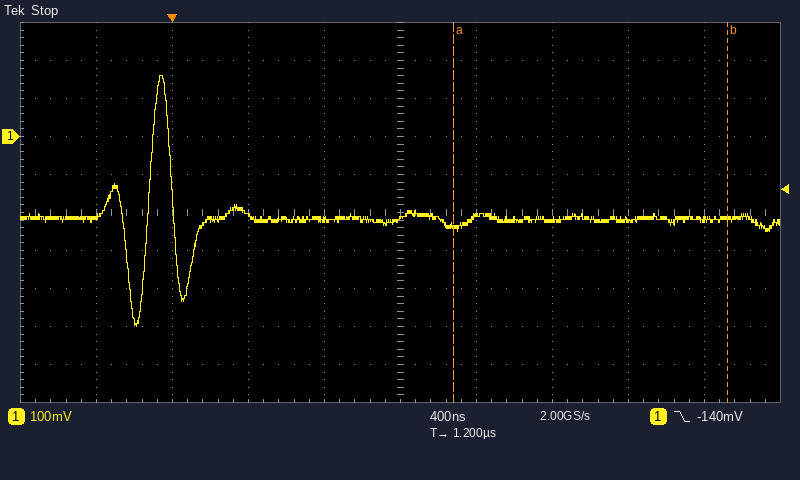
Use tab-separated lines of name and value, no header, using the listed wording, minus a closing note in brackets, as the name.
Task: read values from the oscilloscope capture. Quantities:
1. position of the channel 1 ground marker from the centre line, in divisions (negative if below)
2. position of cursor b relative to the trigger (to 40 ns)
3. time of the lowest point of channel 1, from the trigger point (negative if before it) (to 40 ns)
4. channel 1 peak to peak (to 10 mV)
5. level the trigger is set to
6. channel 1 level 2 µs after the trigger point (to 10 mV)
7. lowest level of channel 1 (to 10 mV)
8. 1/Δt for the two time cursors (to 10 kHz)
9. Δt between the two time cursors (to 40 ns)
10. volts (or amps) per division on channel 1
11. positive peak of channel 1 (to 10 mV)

position of the channel 1 ground marker from the centre line, in divisions	+2.0 div
position of cursor b relative to the trigger	+2.92 µs
time of the lowest point of channel 1, from the trigger point (negative if before it)	-200 ns
channel 1 peak to peak	660 mV
level the trigger is set to	-140 mV
channel 1 level 2 µs after the trigger point	-220 mV
lowest level of channel 1	-500 mV
1/Δt for the two time cursors	690 kHz
Δt between the two time cursors	1.44 µs
volts (or amps) per division on channel 1	100 mV
positive peak of channel 1	160 mV
